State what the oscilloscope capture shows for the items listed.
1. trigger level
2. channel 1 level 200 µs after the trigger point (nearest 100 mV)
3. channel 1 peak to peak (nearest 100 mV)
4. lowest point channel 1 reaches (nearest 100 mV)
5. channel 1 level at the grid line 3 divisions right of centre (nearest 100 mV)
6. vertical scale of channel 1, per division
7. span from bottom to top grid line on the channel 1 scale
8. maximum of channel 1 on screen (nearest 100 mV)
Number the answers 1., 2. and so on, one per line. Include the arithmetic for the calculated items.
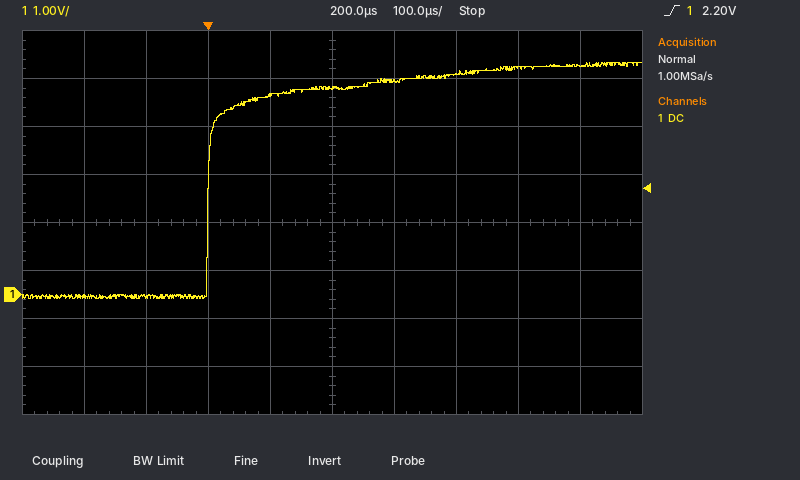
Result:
1. 2.20 V
2. 4.3 V
3. 4.8 V − (-100 mV) = 4.9 V
4. -100 mV
5. 4.7 V
6. 1 V
7. 8 V
8. 4.8 V
